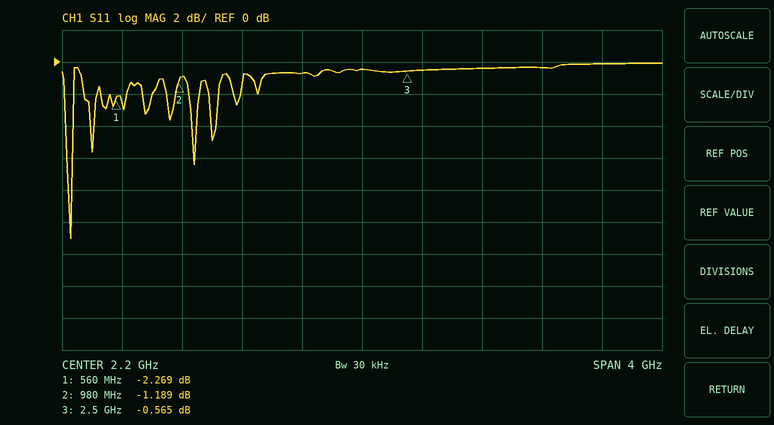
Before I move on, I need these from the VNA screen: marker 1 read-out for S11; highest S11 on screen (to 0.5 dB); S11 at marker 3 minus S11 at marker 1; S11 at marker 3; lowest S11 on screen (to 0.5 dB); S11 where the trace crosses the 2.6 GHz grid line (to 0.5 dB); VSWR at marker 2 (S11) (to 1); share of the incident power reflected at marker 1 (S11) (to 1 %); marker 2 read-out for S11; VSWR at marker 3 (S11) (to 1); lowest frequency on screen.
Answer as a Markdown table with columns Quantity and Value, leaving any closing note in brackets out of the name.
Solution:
| Quantity | Value |
|---|---|
| marker 1 read-out for S11 | -2.269 dB |
| highest S11 on screen | 0.0 dB |
| S11 at marker 3 minus S11 at marker 1 | 1.704 dB |
| S11 at marker 3 | -0.565 dB |
| lowest S11 on screen | -11.0 dB |
| S11 where the trace crosses the 2.6 GHz grid line | -0.5 dB |
| VSWR at marker 2 (S11) | 15 |
| share of the incident power reflected at marker 1 (S11) | 59 % |
| marker 2 read-out for S11 | -1.189 dB |
| VSWR at marker 3 (S11) | 31 |
| lowest frequency on screen | 200 MHz |
